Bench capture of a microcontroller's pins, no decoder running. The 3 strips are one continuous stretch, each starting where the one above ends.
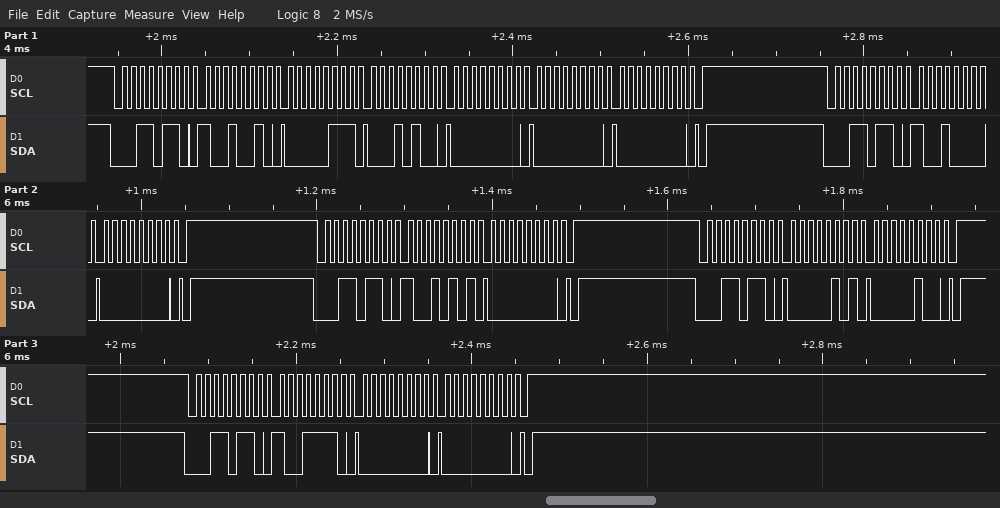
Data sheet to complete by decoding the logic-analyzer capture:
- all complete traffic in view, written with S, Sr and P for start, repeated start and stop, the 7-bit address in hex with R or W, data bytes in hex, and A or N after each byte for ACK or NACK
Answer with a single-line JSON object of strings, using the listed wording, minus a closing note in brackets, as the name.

{"all complete traffic in view, written with S, Sr and P for start, repeated start and stop, the 7-bit address in hex with R or W, data bytes in hex, and A or N after each byte for ACK or NACK": "S 1BW A 92 A 07 A 14 A 00 A 00 A 00 A P S 1BW A 90 A 00 A P S 1BW A 95 A 00 A P S 1BW A 05 A 04 A P S 1BW A 9E A 00 A 00 A P"}
